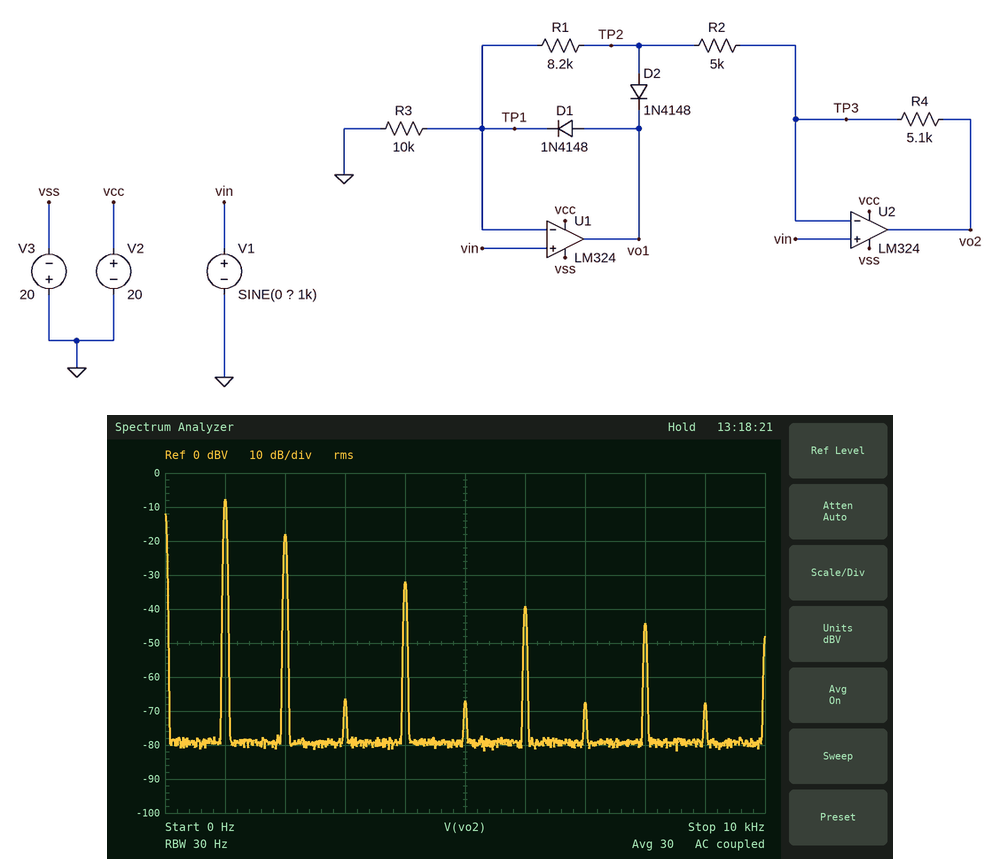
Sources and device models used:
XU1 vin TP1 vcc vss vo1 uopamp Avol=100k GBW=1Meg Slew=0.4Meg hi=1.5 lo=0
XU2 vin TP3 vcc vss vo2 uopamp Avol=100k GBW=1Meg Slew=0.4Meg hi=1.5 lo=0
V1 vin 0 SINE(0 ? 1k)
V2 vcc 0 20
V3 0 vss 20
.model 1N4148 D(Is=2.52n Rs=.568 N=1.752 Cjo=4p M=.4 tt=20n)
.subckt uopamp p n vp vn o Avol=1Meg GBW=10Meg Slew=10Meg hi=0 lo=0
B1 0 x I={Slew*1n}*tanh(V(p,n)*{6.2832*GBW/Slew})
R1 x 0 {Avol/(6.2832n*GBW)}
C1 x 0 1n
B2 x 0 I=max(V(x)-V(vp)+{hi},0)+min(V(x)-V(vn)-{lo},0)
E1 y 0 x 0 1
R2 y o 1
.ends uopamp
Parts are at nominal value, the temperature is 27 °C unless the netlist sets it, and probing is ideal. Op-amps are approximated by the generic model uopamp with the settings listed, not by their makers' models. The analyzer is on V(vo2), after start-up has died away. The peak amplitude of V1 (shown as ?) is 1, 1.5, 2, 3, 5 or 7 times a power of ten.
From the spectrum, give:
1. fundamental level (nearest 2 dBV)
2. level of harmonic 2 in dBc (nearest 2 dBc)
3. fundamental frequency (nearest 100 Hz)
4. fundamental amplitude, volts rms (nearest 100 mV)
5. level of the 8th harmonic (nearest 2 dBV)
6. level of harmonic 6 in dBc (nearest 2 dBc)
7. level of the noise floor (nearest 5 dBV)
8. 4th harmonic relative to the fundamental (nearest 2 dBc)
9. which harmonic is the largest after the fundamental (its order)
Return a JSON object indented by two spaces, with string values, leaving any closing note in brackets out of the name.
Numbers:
{
  "fundamental level": "-8 dBV",
  "level of harmonic 2 in dBc": "-10 dBc",
  "fundamental frequency": "1.0 kHz",
  "fundamental amplitude, volts rms": "400 mV",
  "level of the 8th harmonic": "-44 dBV",
  "level of harmonic 6 in dBc": "-32 dBc",
  "level of the noise floor": "-80 dBV",
  "4th harmonic relative to the fundamental": "-24 dBc",
  "which harmonic is the largest after the fundamental": "2"
}
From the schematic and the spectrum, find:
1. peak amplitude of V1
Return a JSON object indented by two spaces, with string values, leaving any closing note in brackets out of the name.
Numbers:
{
  "peak amplitude of V1": "1 V"
}
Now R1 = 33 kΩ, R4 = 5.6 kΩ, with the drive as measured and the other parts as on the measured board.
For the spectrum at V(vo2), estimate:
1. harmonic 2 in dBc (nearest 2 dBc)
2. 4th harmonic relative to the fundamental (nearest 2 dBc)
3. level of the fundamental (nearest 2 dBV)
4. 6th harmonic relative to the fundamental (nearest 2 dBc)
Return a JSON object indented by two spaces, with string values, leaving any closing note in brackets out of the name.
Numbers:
{
  "harmonic 2 in dBc": "0 dBc",
  "4th harmonic relative to the fundamental": "-14 dBc",
  "level of the fundamental": "-4 dBV",
  "6th harmonic relative to the fundamental": "-22 dBc"
}
